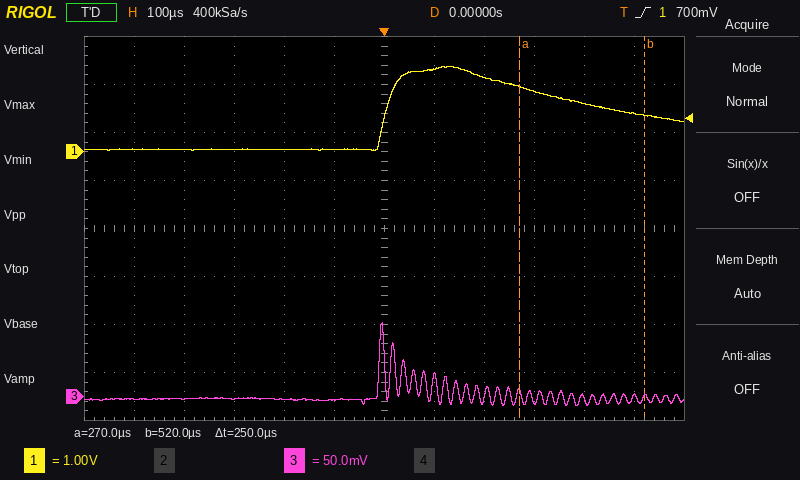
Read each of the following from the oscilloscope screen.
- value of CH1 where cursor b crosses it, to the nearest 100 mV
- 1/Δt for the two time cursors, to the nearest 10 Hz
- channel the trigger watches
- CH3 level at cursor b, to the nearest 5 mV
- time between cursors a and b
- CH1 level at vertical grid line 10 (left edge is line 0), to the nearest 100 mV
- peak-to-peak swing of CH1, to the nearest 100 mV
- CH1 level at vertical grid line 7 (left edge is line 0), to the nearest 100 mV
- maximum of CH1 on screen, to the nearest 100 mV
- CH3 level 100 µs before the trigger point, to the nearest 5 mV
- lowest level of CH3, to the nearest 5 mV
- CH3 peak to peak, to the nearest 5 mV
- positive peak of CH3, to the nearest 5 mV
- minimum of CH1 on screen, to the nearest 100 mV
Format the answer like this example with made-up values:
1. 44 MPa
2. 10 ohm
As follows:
1. 800 mV
2. 4.00 kHz
3. CH1
4. 0 mV
5. 250 µs
6. 1.0 V
7. 1.8 V
8. 1.7 V
9. 1.8 V
10. -5 mV
11. -10 mV
12. 85 mV
13. 75 mV
14. 0.0 V
